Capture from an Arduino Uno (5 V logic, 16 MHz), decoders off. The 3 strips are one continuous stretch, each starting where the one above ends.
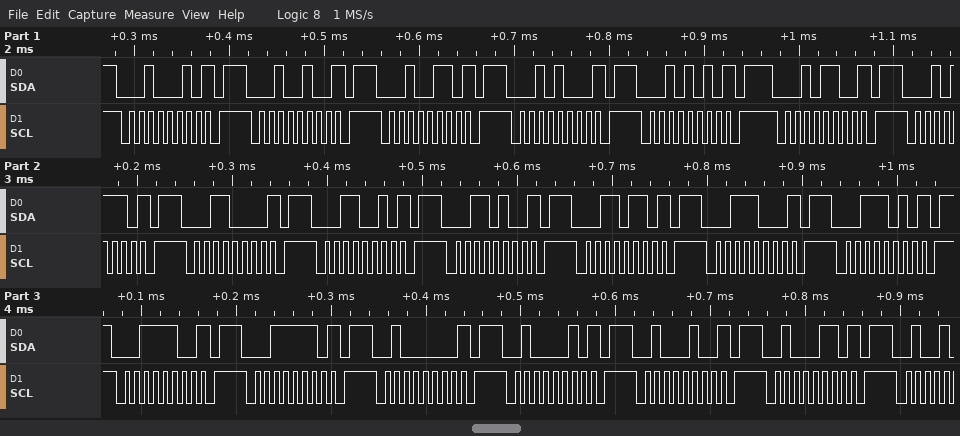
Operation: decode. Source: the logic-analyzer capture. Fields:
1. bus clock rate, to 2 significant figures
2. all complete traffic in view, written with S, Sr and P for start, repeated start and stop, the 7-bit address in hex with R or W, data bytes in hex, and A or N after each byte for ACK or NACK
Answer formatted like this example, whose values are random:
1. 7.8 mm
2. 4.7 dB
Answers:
1. 100 kHz
2. S 11W N P S 12W N P S 13W N P S 14W N P S 15W N P S 16W N P S 17W N P S 18W N P S 19W N P S 1AW N P S 1BW N P S 1CW N P S 1DW N P S 1EW N P S 1FW N P S 20W N P S 21W N P S 22W N P S 23W N P
